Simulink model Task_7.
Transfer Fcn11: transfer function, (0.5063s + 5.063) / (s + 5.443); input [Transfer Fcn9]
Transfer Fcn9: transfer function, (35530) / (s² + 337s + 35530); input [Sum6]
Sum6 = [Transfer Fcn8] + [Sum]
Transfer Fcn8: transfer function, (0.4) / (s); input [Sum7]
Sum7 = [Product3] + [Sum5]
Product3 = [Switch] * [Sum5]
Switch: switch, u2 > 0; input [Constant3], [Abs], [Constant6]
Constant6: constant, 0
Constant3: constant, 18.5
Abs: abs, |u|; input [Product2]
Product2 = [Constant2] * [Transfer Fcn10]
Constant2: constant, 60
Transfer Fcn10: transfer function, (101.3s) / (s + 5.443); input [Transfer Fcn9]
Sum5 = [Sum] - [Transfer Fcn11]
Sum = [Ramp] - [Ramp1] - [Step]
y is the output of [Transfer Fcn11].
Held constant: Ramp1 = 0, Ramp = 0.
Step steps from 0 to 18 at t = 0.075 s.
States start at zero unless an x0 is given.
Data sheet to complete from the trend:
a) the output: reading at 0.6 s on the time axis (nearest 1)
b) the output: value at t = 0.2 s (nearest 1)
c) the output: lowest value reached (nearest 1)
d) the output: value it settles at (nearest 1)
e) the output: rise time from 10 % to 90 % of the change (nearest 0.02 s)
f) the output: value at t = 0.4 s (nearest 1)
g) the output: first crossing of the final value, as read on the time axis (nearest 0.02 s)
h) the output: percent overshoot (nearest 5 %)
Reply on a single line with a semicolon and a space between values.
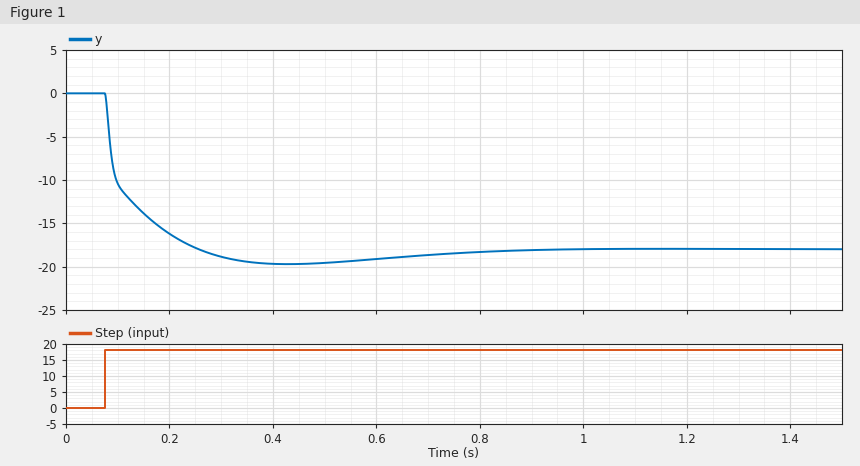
-19; -16; -20; -18; 0.12 s; -20; 0.26 s; 10 %
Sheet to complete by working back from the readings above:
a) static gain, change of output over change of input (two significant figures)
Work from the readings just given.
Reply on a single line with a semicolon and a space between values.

-1.0
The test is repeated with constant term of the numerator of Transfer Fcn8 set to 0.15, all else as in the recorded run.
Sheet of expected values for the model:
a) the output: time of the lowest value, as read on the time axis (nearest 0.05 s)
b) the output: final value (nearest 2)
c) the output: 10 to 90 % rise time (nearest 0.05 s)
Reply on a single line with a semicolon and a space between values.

0.65 s; -18; 0.20 s
